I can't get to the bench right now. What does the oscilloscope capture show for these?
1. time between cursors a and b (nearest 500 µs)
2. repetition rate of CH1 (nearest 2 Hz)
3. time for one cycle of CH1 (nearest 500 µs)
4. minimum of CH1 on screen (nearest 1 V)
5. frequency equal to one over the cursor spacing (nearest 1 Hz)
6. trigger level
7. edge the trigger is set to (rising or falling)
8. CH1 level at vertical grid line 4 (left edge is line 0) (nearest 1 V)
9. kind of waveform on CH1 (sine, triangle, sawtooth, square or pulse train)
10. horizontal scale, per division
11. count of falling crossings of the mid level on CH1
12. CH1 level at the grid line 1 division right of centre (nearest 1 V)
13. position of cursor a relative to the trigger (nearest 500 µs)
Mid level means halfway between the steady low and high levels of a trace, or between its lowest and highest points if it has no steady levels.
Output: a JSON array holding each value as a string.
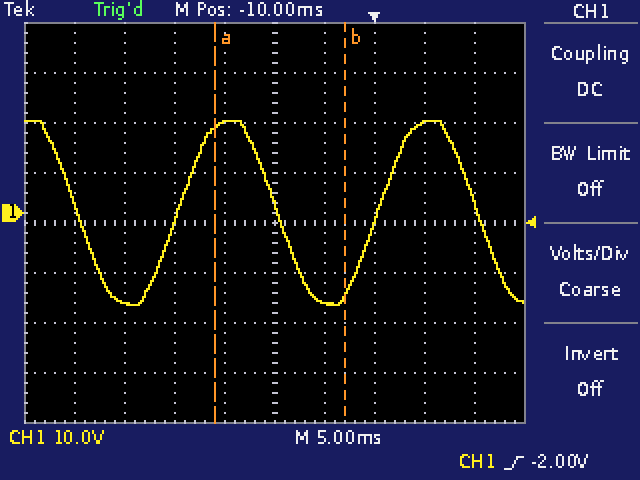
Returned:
["13.0 ms", "50 Hz", "20.0 ms", "-18 V", "77 Hz", "-2.00 V", "rising", "18 V", "sine", "5 ms", "3", "-18 V", "-16.0 ms"]
